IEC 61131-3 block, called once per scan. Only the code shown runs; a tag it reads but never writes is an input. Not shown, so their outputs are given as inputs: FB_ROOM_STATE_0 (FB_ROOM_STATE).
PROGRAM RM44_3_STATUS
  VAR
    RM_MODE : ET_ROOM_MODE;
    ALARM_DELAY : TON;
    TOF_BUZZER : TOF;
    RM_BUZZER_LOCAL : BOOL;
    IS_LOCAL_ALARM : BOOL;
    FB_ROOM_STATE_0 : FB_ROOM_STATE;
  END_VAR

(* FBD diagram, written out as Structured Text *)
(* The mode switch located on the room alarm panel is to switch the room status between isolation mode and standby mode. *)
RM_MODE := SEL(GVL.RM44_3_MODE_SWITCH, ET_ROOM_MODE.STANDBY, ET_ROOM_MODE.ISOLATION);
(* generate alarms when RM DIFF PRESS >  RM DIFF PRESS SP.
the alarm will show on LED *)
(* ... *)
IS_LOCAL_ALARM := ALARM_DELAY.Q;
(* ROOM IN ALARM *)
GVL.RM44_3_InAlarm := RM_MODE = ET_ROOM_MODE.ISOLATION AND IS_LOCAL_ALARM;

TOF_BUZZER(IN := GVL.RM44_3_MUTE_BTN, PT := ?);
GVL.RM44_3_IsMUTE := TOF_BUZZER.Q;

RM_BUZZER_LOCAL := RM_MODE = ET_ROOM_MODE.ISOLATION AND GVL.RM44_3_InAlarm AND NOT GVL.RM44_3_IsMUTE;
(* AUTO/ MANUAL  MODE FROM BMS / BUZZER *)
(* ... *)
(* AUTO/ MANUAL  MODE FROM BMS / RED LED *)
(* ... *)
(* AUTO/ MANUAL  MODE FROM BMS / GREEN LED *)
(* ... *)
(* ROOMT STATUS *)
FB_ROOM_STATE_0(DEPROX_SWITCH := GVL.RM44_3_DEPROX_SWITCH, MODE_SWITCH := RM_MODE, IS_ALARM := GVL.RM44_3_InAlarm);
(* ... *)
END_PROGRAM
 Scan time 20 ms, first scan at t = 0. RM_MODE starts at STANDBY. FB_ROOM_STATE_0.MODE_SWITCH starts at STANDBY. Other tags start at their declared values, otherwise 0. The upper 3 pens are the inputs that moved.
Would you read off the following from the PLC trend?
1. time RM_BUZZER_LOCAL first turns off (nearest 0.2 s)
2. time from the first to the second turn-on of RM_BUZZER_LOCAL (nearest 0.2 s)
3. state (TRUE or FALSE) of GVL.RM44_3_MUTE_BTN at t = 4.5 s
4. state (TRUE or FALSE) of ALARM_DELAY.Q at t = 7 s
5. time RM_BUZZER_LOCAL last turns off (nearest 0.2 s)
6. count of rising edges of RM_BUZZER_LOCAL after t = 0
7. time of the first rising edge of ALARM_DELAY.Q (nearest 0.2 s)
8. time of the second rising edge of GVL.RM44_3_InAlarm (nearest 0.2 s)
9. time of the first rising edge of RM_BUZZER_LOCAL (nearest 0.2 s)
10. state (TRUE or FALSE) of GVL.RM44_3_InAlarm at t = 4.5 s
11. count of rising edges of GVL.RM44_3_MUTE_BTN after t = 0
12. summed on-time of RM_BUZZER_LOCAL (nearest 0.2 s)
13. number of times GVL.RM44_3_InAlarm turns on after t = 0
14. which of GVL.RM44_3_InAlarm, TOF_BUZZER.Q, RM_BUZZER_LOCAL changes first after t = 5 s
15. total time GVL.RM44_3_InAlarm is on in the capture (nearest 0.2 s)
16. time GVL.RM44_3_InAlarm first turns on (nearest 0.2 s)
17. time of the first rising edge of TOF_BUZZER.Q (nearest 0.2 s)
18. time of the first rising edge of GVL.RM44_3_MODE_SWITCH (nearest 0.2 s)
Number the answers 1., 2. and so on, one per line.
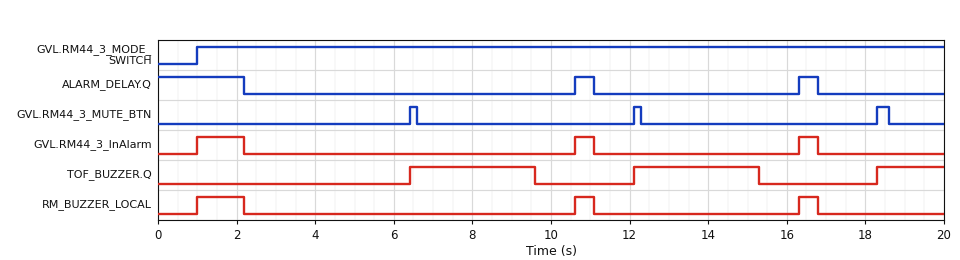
1. 2.2 s
2. 9.6 s
3. FALSE
4. FALSE
5. 16.8 s
6. 3
7. 10.6 s
8. 10.6 s
9. 1.0 s
10. FALSE
11. 3
12. 2.2 s
13. 3
14. TOF_BUZZER.Q
15. 2.2 s
16. 1.0 s
17. 6.4 s
18. 1.0 s
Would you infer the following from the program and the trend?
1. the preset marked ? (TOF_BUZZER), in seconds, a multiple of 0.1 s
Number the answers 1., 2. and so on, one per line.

1. 3.0 s
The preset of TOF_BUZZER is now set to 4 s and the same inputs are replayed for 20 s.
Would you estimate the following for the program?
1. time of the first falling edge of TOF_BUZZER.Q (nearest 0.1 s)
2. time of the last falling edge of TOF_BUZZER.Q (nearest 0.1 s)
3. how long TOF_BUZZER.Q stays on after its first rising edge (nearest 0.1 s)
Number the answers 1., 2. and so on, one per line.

1. 10.6 s
2. 16.3 s
3. 4.2 s
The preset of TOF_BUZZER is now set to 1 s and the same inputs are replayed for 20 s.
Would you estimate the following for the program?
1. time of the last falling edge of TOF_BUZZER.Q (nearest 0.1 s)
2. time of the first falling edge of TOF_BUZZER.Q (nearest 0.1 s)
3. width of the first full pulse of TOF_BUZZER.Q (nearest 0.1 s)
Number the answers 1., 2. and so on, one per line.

1. 19.6 s
2. 7.6 s
3. 1.2 s
